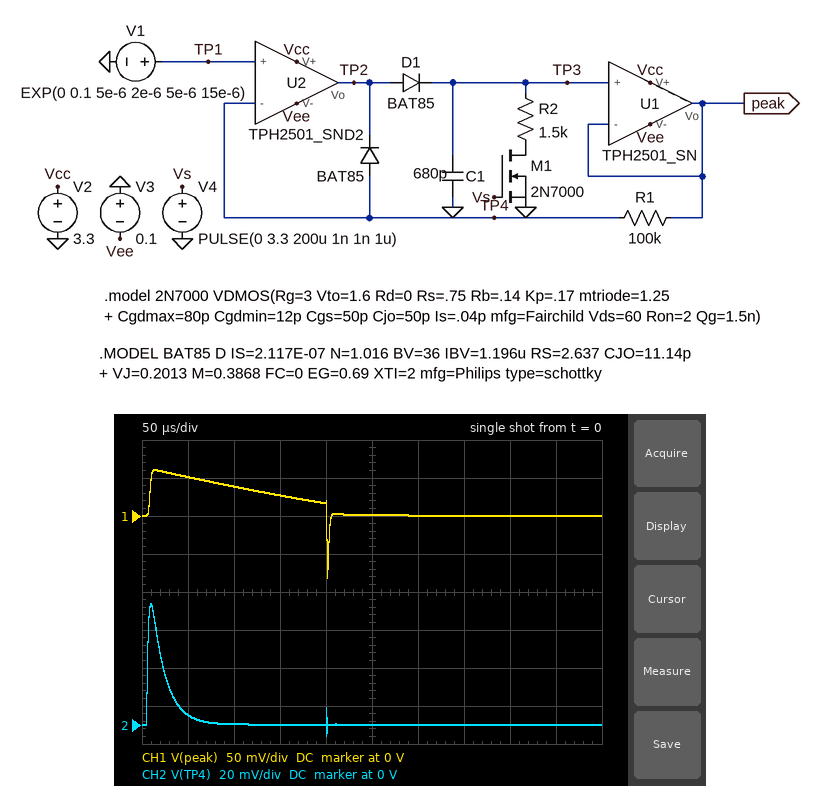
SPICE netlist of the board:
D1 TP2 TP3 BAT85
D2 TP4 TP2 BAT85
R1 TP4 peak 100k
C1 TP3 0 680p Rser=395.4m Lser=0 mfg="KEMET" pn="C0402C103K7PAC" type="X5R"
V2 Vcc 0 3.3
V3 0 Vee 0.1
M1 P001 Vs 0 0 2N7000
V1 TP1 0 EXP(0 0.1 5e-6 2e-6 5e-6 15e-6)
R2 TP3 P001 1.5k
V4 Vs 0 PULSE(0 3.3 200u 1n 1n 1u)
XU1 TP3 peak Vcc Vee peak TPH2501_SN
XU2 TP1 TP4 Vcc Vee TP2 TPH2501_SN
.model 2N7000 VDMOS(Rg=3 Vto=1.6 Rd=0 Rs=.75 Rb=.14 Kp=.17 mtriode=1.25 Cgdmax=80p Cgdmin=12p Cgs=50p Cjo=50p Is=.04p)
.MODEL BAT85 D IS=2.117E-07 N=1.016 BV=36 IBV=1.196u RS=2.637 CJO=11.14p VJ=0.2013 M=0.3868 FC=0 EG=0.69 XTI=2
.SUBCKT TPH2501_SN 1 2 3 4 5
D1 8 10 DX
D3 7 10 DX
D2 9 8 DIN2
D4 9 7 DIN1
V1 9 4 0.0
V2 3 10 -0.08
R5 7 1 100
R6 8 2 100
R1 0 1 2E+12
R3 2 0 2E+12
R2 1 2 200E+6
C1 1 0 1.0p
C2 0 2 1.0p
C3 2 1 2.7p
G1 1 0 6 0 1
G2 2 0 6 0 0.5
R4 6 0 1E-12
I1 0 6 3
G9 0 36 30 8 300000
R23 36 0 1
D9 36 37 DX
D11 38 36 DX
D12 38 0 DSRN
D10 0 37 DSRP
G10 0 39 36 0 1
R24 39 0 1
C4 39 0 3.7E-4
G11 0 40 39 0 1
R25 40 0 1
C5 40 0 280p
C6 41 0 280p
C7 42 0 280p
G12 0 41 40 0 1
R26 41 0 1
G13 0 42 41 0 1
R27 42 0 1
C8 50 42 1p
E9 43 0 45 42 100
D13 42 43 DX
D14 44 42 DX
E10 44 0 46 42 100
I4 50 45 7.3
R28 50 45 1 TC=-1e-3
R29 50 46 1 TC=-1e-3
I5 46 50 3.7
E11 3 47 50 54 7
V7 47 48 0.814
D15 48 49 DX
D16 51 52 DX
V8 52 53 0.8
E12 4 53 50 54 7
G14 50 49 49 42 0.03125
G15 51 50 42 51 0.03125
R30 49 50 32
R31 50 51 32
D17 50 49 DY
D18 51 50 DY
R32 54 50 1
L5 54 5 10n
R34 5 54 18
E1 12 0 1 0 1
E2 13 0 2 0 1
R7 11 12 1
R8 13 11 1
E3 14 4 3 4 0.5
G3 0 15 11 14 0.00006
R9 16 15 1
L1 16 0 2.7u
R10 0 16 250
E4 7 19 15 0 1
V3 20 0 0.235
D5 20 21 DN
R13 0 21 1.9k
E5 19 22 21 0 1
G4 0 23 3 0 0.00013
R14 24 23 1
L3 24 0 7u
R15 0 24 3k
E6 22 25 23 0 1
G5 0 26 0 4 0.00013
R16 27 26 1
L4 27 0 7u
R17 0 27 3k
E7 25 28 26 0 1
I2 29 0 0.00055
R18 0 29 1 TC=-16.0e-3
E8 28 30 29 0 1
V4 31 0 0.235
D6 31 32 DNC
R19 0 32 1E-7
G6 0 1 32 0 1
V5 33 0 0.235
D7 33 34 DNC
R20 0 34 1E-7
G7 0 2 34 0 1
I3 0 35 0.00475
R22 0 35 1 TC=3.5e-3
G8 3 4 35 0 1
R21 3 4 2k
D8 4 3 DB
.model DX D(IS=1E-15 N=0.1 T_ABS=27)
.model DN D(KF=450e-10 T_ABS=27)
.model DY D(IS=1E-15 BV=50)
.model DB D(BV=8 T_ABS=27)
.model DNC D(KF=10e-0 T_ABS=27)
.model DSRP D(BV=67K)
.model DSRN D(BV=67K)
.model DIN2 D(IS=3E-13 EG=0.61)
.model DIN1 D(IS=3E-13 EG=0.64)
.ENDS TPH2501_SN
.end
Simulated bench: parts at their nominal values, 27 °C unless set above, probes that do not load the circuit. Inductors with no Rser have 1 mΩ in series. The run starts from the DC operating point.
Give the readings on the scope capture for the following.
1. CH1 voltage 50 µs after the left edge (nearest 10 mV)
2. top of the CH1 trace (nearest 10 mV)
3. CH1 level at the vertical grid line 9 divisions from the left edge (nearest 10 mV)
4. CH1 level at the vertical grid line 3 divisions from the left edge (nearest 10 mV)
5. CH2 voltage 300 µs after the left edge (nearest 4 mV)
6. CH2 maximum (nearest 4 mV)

50 mV
60 mV
0 V
30 mV
0 V
64 mV
